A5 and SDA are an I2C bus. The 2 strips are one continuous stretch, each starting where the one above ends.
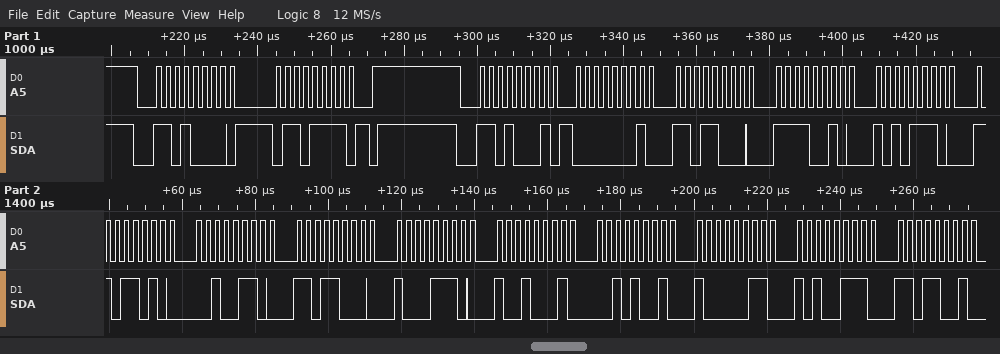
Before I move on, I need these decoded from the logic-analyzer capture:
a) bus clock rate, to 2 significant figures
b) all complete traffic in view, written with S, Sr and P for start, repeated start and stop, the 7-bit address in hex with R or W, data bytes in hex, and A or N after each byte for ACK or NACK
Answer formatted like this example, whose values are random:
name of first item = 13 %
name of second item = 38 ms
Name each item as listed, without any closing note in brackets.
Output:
bus clock rate, to 2 significant figures = 400 kHz
all complete traffic in view, written with S, Sr and P for start, repeated start and stop, the 7-bit address in hex with R or W, data bytes in hex, and A or N after each byte for ACK or NACK = S 68W A 6F A P S 68R A 01 A D8 A F2 A AE A DA A 26 A D8 A 8E A 91 A 29 A 83 A A7 A D9 A
